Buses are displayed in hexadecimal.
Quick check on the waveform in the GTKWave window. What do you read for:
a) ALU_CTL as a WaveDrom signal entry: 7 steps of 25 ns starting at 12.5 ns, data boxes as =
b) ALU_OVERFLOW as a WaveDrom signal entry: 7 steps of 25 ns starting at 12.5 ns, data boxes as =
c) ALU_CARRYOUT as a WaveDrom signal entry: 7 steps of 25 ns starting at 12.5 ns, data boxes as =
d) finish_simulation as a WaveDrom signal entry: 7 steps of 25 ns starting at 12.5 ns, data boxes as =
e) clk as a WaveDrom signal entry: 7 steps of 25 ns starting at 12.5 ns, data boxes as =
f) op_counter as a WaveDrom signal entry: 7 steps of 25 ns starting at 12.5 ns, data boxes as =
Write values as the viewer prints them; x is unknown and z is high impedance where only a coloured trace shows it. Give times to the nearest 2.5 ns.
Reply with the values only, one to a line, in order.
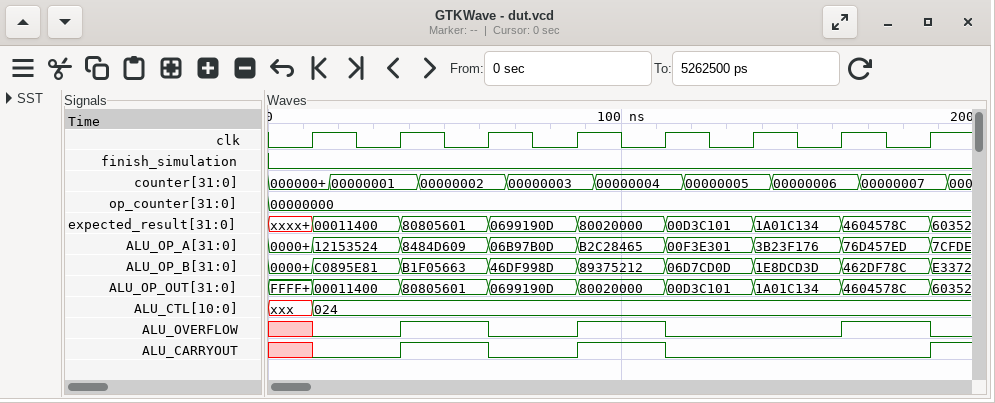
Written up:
{name: 'ALU_CTL', wave: '=......', data: '024'}
{name: 'ALU_OVERFLOW', wave: '01010.1'}
{name: 'ALU_CARRYOUT', wave: '01010..'}
{name: 'finish_simulation', wave: '0......'}
{name: 'clk', wave: 'p......'}
{name: 'op_counter', wave: '=......', data: '00000000'}
